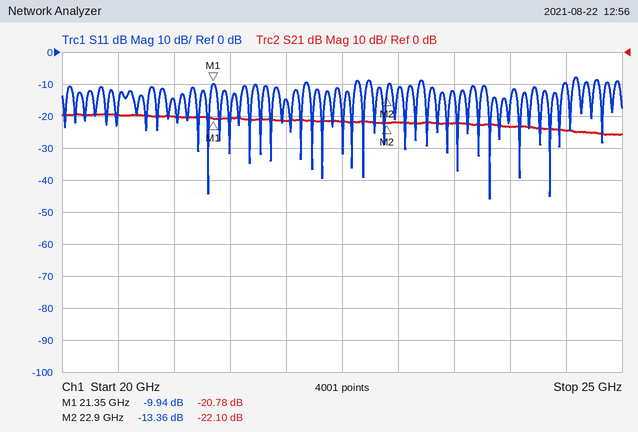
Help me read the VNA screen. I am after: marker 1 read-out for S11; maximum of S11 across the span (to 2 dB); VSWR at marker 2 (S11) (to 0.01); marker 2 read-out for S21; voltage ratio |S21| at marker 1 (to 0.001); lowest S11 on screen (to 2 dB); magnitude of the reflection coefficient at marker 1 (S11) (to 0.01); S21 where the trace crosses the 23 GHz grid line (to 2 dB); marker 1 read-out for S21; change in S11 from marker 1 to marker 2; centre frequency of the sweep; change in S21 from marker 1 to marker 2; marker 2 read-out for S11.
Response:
-9.94 dB
-8 dB
1.55
-22.10 dB
0.091
-46 dB
0.32
-22 dB
-20.78 dB
-3.42 dB
22.5 GHz
-1.32 dB
-13.36 dB
